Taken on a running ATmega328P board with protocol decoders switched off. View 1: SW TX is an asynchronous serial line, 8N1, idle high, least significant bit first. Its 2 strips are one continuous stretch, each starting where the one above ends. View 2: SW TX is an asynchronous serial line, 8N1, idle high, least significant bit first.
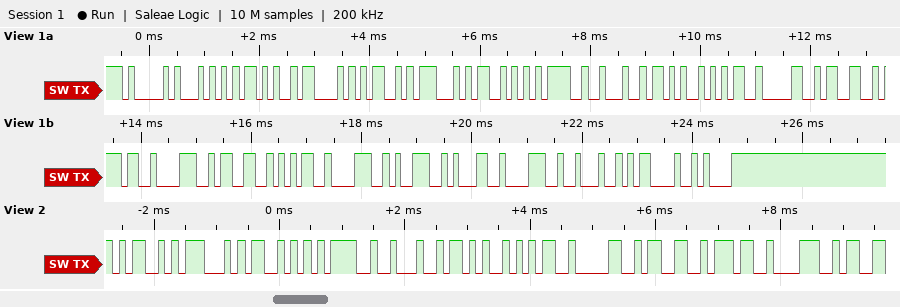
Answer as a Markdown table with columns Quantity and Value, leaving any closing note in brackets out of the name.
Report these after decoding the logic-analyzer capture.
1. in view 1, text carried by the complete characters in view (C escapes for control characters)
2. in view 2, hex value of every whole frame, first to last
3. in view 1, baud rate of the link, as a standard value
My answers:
| Quantity | Value |
|---|---|
| in view 1, text carried by the complete characters in view | "AT+CMGS=\"+50378358918\"\r\n" |
| in view 2, hex value of every whole frame, first to last | 4D 47 53 3D 22 2B 35 30 33 37 38 |
| in view 1, baud rate of the link, as a standard value | 9600 baud |
